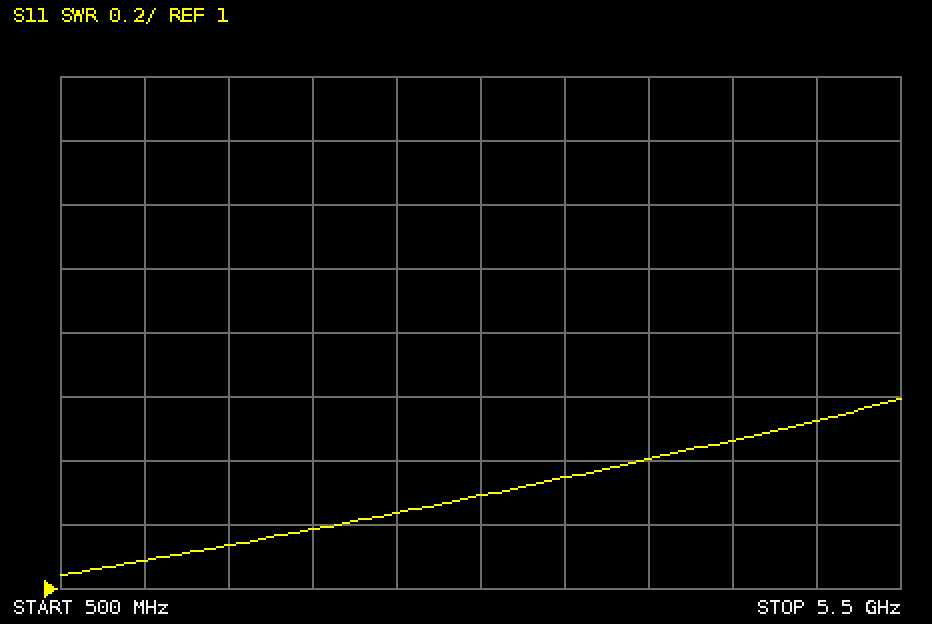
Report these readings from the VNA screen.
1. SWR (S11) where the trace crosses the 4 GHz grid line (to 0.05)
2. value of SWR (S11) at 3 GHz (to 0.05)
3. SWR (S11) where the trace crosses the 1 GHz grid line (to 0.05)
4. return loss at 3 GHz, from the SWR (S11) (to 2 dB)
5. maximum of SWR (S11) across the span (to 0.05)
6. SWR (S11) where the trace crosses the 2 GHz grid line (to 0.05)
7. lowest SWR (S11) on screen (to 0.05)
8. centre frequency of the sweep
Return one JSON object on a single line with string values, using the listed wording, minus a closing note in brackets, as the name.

{"SWR (S11) where the trace crosses the 4 GHz grid line": "1.40", "value of SWR (S11) at 3 GHz": "1.30", "SWR (S11) where the trace crosses the 1 GHz grid line": "1.10", "return loss at 3 GHz, from the SWR (S11)": "18 dB", "maximum of SWR (S11) across the span": "1.60", "SWR (S11) where the trace crosses the 2 GHz grid line": "1.20", "lowest SWR (S11) on screen": "1.05", "centre frequency of the sweep": "3 GHz"}
